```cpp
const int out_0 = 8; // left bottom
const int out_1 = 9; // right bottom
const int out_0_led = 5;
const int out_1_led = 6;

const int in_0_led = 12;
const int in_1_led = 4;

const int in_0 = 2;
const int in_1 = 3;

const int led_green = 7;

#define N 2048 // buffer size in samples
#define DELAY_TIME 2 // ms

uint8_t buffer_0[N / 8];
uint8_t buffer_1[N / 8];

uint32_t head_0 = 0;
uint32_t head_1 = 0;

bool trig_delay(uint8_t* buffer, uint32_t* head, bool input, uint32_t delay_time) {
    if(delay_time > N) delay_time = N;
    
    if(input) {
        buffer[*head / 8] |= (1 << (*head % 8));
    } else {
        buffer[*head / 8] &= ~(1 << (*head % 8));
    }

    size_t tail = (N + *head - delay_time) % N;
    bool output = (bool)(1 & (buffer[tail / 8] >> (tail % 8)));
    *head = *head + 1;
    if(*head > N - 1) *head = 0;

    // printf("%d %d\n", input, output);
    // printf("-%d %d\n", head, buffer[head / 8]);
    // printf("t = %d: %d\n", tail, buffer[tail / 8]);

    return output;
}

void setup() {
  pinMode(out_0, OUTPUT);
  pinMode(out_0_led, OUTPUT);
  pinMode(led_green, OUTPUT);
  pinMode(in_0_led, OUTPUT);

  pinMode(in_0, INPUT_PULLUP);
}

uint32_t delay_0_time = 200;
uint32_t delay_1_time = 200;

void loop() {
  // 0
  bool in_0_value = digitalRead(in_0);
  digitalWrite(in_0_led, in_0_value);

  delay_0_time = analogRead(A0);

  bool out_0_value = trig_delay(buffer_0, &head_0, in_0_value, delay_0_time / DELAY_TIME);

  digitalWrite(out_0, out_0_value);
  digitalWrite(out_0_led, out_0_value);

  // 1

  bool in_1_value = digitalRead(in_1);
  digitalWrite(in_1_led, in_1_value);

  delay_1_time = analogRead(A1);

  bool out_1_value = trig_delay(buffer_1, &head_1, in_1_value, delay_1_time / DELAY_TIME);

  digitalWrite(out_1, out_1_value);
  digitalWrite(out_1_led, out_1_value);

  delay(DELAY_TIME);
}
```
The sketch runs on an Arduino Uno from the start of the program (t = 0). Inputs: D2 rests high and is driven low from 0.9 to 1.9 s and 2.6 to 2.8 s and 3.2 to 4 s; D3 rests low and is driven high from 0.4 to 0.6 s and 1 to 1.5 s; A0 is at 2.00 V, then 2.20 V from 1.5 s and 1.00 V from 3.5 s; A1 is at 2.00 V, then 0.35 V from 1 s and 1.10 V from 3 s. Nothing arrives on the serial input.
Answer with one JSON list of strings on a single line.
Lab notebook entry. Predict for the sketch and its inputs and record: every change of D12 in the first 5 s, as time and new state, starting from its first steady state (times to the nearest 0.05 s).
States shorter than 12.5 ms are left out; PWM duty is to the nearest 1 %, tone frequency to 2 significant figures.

["0 s high; 0.9 s low; 1.9 s high; 2.6 s low; 2.8 s high; 3.2 s low; 4 s high"]
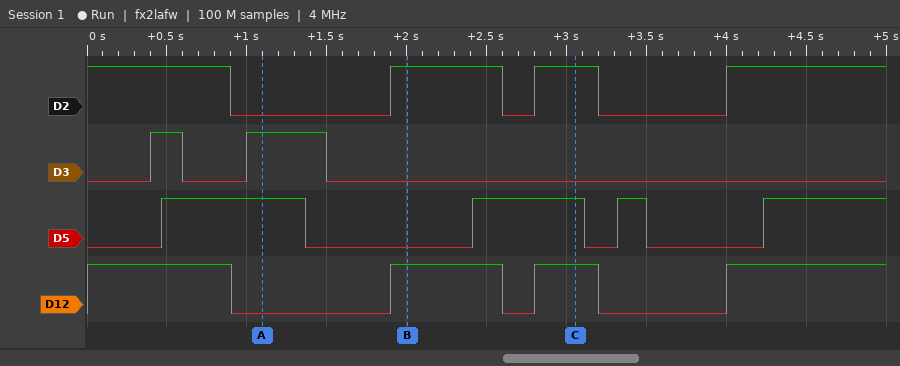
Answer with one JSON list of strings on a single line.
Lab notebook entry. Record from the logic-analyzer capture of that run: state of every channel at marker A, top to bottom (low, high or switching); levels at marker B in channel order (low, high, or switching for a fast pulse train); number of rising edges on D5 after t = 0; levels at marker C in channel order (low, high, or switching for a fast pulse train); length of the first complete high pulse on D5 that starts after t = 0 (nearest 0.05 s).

["D2 low, D3 high, D5 high, D12 low", "D2 high, D3 low, D5 low, D12 high", "4", "D2 high, D3 low, D5 high, D12 high", "0.90 s"]
